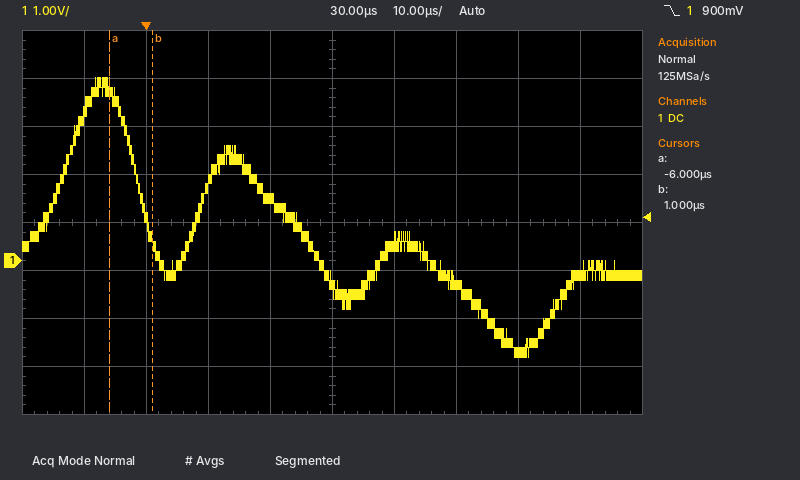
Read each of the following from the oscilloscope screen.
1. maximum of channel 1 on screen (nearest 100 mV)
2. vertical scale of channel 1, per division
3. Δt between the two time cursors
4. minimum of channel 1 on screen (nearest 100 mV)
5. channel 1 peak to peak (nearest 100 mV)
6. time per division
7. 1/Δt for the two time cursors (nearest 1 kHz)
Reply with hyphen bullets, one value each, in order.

- 3.8 V
- 1 V
- 7 µs
- -2.0 V
- 5.8 V
- 10 µs
- 143 kHz
